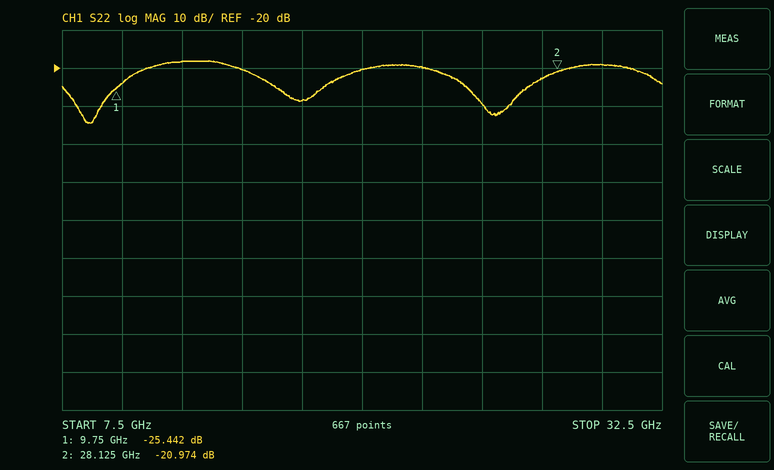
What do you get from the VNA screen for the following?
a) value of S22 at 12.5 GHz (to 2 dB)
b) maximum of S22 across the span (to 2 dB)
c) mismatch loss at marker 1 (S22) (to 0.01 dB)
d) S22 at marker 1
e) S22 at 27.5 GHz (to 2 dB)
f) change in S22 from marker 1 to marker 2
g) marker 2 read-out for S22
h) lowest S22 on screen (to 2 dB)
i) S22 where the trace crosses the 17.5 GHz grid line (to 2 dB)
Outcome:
-18 dB
-18 dB
0.01 dB
-25.442 dB
-22 dB
4.468 dB
-20.974 dB
-34 dB
-28 dB
